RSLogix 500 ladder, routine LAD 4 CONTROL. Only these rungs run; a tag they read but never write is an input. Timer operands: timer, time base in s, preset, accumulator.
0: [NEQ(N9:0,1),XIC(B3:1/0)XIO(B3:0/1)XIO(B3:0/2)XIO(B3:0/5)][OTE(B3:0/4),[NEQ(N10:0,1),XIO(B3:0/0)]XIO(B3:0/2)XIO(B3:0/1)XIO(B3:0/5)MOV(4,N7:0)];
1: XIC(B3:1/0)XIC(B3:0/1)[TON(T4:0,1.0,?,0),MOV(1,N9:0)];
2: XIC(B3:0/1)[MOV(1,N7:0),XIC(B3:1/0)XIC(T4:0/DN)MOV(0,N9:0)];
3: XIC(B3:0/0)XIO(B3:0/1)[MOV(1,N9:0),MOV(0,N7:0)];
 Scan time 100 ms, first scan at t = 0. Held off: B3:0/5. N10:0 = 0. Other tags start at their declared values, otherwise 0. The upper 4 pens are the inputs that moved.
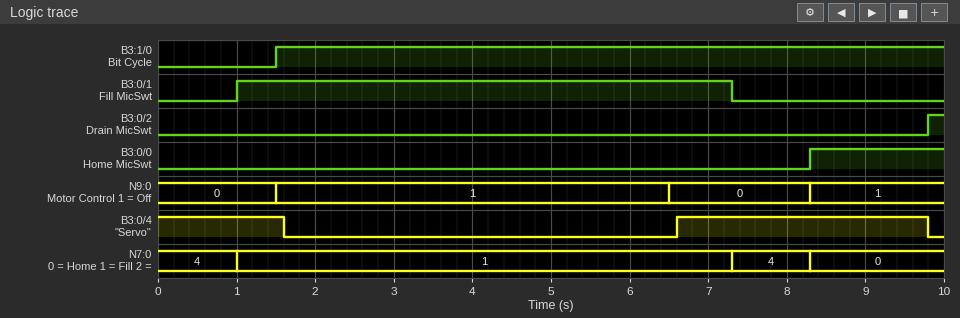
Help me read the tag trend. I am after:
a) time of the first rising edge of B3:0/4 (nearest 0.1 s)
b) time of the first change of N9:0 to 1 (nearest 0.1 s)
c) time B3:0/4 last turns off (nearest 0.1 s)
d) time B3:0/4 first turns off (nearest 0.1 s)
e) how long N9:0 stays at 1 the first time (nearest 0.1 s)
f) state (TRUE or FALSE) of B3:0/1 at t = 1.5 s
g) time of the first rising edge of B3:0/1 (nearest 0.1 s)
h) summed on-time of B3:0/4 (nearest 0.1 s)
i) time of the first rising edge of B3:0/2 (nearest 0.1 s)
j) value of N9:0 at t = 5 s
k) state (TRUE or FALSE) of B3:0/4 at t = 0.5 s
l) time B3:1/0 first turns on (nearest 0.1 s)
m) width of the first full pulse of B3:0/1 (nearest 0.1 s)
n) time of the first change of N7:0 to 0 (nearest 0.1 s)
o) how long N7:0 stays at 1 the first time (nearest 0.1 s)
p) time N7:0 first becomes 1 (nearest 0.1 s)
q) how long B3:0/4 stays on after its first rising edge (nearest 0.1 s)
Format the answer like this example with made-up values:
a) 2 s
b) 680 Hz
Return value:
a) 6.6 s
b) 1.5 s
c) 9.8 s
d) 1.6 s
e) 5.0 s
f) TRUE
g) 1.0 s
h) 4.8 s
i) 9.8 s
j) 1
k) TRUE
l) 1.5 s
m) 6.3 s
n) 8.3 s
o) 6.3 s
p) 1.0 s
q) 3.2 s
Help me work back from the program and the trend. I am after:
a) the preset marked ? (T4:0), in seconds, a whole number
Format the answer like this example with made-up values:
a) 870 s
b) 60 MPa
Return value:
a) 5 s
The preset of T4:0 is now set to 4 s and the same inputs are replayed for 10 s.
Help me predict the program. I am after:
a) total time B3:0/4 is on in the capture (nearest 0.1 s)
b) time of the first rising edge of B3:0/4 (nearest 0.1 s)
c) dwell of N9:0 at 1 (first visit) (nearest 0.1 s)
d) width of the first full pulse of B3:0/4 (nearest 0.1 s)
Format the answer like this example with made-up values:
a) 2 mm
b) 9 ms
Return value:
a) 5.8 s
b) 5.6 s
c) 4.0 s
d) 4.2 s
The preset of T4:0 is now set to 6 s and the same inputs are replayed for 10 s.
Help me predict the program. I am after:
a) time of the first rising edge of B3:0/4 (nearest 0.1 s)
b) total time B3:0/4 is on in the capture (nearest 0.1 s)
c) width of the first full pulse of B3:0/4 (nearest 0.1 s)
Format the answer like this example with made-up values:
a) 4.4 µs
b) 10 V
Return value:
a) 7.3 s
b) 4.1 s
c) 2.5 s
